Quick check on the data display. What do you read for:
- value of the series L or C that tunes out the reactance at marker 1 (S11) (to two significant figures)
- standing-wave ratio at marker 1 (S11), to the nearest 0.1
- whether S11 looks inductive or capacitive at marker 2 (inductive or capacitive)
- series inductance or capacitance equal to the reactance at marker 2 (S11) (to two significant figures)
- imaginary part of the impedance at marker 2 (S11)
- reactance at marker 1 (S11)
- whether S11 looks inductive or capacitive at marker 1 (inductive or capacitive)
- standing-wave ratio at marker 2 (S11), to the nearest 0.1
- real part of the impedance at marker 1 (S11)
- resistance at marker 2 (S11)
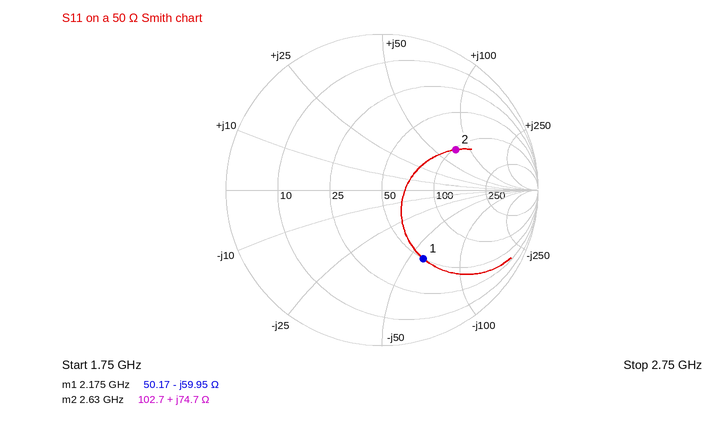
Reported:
4.4 nH
3.1
inductive
4.5 nH
+74.7 Ω
-59.95 Ω
capacitive
3.3
50.17 Ω
102.7 Ω
